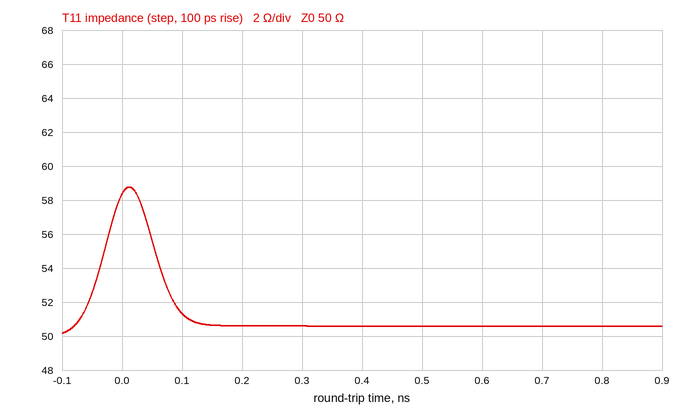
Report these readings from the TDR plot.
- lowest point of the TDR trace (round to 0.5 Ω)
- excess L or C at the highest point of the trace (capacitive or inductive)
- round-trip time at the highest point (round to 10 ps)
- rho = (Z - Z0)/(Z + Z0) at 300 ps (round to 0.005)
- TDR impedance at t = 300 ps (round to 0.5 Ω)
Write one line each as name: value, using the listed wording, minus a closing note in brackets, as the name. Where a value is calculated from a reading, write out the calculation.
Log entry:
lowest point of the TDR trace: 50.0 Ω
excess L or C at the highest point of the trace: inductive
round-trip time at the highest point: 10 ps
rho = (Z - Z0)/(Z + Z0) at 300 ps: (50.5 − 50)/(50.5 + 50) ≈ +0.005
TDR impedance at t = 300 ps: 50.5 Ω
